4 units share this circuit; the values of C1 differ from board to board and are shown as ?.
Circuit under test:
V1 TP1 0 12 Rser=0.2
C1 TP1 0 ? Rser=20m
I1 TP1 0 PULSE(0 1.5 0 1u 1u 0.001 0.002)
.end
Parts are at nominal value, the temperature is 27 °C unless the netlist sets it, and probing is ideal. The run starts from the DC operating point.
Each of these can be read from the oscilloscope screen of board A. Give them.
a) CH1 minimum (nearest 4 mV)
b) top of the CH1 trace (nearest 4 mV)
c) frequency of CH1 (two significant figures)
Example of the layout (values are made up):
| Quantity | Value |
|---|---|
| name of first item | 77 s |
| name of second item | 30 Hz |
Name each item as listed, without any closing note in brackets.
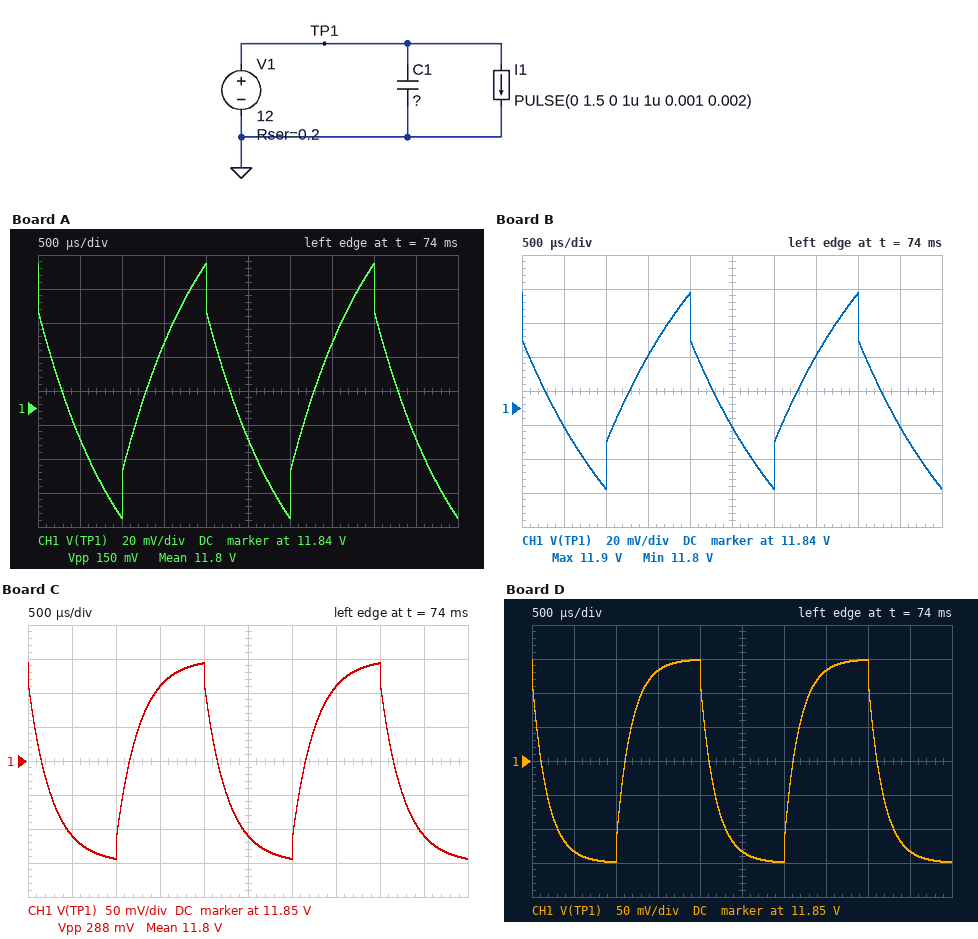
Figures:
| Quantity | Value |
|---|---|
| CH1 minimum | 11.776 V |
| top of the CH1 trace | 11.924 V |
| frequency of CH1 | 500 Hz |
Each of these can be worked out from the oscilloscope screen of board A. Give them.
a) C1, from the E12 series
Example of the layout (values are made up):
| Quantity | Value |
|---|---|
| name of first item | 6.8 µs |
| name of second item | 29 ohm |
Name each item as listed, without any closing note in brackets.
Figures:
| Quantity | Value |
|---|---|
| C1, from the E12 series | 4.7 mF |
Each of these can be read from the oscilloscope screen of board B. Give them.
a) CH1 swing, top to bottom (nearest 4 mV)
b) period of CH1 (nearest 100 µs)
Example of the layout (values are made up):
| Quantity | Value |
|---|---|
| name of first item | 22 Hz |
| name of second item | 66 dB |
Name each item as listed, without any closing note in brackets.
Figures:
| Quantity | Value |
|---|---|
| CH1 swing, top to bottom | 116 mV |
| period of CH1 | 2.0 ms |
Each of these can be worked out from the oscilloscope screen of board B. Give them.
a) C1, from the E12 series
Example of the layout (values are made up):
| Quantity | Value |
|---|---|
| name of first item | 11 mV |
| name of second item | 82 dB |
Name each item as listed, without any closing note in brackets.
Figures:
| Quantity | Value |
|---|---|
| C1, from the E12 series | 6.8 mF |
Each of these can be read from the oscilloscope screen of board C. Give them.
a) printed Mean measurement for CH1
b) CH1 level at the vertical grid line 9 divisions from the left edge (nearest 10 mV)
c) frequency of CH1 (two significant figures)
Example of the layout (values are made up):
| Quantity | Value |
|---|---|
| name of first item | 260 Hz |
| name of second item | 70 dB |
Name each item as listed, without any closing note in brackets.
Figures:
| Quantity | Value |
|---|---|
| printed Mean measurement for CH1 | 11.8 V |
| CH1 level at the vertical grid line 9 divisions from the left edge | 11.74 V |
| frequency of CH1 | 500 Hz |
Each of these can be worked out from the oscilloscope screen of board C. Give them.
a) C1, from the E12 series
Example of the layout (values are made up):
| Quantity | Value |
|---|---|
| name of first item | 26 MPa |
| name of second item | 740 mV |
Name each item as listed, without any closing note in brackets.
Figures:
| Quantity | Value |
|---|---|
| C1, from the E12 series | 1.2 mF |
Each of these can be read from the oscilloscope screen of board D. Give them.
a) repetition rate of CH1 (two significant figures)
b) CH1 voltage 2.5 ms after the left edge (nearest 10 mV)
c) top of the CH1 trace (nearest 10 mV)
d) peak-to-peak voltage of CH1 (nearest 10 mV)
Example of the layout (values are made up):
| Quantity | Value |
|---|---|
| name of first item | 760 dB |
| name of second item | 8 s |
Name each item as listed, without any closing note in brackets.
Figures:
| Quantity | Value |
|---|---|
| repetition rate of CH1 | 500 Hz |
| CH1 voltage 2.5 ms after the left edge | 11.72 V |
| top of the CH1 trace | 12.00 V |
| peak-to-peak voltage of CH1 | 300 mV |
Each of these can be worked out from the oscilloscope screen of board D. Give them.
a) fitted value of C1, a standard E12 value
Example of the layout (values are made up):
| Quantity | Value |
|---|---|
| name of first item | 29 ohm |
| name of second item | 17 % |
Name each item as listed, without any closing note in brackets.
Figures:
| Quantity | Value |
|---|---|
| fitted value of C1, a standard E12 value | 820 µF |
